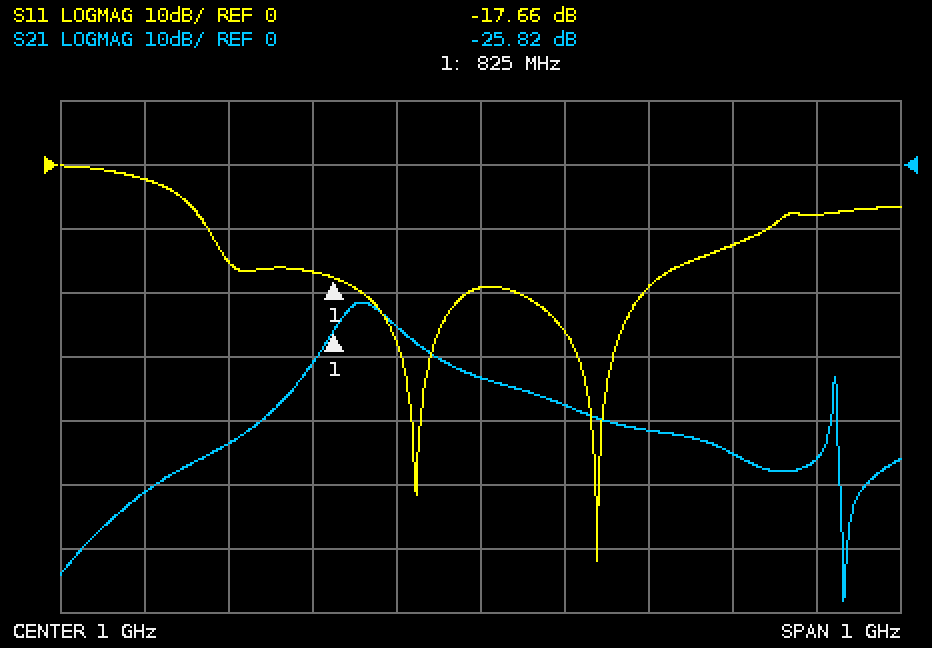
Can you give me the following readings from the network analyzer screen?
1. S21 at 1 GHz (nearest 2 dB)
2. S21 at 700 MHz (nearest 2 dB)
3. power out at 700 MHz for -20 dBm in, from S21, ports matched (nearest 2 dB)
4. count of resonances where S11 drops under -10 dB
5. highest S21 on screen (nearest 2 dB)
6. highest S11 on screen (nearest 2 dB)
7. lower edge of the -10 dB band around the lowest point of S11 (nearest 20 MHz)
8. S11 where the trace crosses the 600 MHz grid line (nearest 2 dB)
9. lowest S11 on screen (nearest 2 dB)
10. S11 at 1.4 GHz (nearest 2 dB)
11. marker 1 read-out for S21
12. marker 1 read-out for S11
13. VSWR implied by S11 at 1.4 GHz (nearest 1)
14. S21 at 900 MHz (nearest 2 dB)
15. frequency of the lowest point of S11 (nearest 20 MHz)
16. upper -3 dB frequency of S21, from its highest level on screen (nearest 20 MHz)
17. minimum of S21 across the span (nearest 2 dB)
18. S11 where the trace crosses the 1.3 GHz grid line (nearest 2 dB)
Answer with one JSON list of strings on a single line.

["-34 dB", "-44 dB", "-64 dBm", "2", "-22 dB", "0 dB", "680 MHz", "-2 dB", "-62 dB", "-8 dB", "-25.82 dB", "-17.66 dB", "2", "-26 dB", "1.14 GHz", "900 MHz", "-68 dB", "-12 dB"]
